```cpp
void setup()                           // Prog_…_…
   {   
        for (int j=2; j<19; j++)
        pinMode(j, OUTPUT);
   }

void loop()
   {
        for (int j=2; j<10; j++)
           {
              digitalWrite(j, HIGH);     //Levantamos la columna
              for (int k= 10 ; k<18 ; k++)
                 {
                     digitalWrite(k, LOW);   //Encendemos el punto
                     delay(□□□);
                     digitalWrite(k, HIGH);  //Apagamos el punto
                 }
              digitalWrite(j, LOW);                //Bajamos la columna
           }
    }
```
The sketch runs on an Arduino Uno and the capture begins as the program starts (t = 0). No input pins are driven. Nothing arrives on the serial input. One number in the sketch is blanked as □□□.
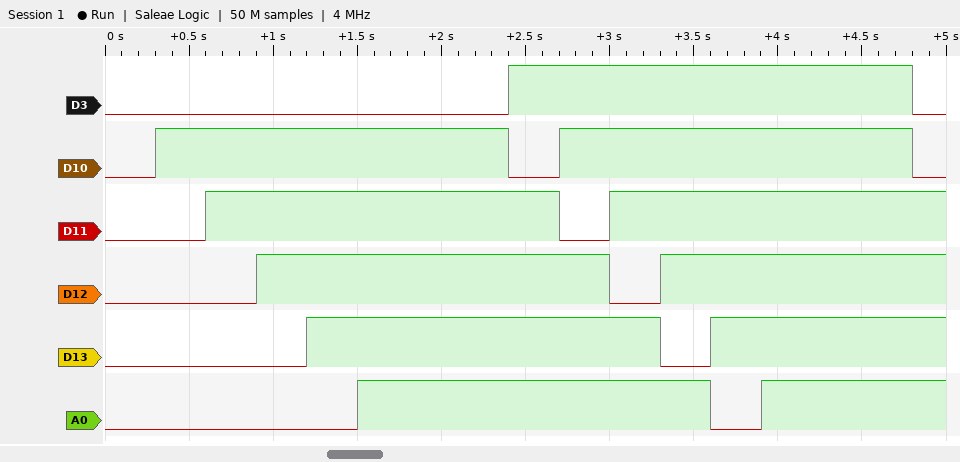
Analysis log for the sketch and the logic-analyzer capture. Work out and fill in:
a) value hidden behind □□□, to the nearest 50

300
